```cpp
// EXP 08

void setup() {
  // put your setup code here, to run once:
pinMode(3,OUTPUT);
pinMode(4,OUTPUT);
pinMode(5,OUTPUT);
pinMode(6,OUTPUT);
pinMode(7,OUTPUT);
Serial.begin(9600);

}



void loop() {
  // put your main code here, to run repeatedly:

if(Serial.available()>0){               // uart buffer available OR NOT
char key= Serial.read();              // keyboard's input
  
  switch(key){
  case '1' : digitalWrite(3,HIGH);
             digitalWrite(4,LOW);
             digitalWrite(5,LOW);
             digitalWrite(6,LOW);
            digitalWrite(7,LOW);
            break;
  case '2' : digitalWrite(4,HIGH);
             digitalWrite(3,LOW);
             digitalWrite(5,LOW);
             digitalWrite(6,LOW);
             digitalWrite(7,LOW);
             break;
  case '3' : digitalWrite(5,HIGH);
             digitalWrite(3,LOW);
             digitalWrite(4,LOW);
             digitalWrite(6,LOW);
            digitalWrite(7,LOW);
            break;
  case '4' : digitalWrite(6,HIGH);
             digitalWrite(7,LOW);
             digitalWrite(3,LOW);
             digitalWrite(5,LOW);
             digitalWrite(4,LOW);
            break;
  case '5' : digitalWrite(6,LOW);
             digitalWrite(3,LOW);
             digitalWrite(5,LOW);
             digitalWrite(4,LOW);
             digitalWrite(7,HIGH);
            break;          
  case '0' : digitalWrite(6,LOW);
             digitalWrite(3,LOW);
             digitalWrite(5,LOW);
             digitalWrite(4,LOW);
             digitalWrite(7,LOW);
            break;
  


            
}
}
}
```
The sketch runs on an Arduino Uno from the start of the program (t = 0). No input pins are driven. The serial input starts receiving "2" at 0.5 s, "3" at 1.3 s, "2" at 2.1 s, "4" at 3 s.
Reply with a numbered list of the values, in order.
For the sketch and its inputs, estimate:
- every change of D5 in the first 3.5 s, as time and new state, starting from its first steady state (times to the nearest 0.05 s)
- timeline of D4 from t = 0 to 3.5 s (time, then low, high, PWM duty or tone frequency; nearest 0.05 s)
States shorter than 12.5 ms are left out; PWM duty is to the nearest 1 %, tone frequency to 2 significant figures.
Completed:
1. 0 s low; 1.3 s high; 2.1 s low
2. 0 s low; 0.5 s high; 1.3 s low; 2.1 s high; 3 s low
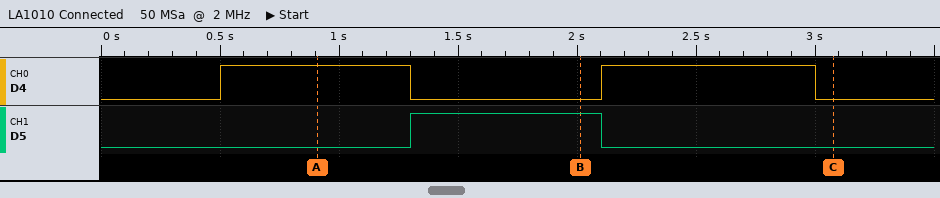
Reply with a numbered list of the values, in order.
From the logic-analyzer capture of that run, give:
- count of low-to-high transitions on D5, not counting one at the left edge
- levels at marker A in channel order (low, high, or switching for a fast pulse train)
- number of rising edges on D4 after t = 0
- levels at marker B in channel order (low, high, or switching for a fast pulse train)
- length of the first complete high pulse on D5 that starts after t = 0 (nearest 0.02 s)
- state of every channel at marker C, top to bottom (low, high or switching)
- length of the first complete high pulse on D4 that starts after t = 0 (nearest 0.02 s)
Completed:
1. 1
2. D4 high, D5 low
3. 2
4. D4 low, D5 high
5. 0.80 s
6. D4 low, D5 low
7. 0.80 s
